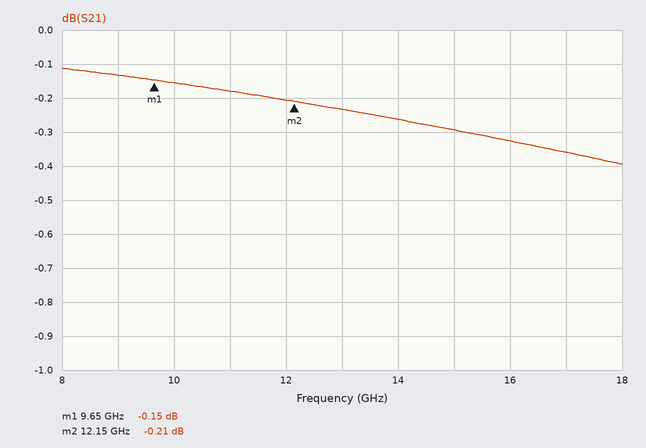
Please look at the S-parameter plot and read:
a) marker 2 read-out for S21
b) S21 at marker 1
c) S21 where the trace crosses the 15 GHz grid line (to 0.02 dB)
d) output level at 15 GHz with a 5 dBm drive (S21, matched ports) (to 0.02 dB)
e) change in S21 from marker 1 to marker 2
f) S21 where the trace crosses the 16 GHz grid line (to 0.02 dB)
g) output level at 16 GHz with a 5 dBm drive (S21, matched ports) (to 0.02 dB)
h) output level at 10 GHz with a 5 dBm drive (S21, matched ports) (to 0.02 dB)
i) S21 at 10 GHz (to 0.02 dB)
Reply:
-0.21 dB
-0.15 dB
-0.30 dB
4.70 dBm
-0.06 dB
-0.32 dB
4.68 dBm
4.84 dBm
-0.16 dB
